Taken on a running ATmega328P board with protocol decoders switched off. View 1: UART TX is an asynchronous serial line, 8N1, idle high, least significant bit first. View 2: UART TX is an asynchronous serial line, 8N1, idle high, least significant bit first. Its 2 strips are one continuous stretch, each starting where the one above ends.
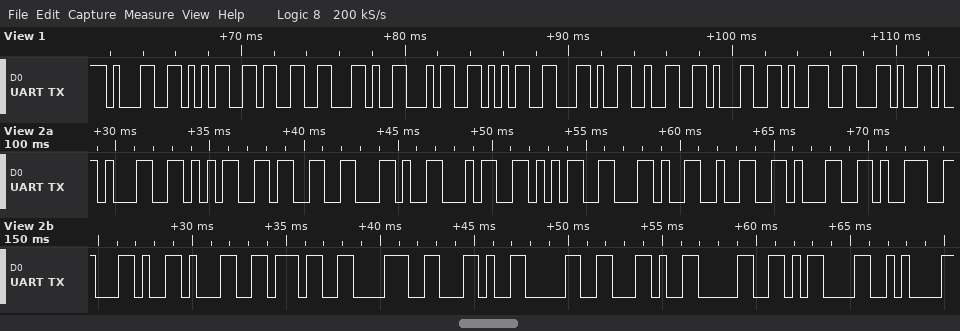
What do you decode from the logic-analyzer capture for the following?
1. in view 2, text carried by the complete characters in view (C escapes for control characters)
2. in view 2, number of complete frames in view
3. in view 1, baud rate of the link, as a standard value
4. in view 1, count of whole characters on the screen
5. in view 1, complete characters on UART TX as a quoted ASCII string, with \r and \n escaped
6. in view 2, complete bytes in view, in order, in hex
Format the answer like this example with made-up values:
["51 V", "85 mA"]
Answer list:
["\"153,45,219,178,0,0\\r\\n\"", "20", "2400 baud", "11", "\"153,45,219,\"", "31 35 33 2C 34 35 2C 32 31 39 2C 31 37 38 2C 30 2C 30 0D 0A"]
